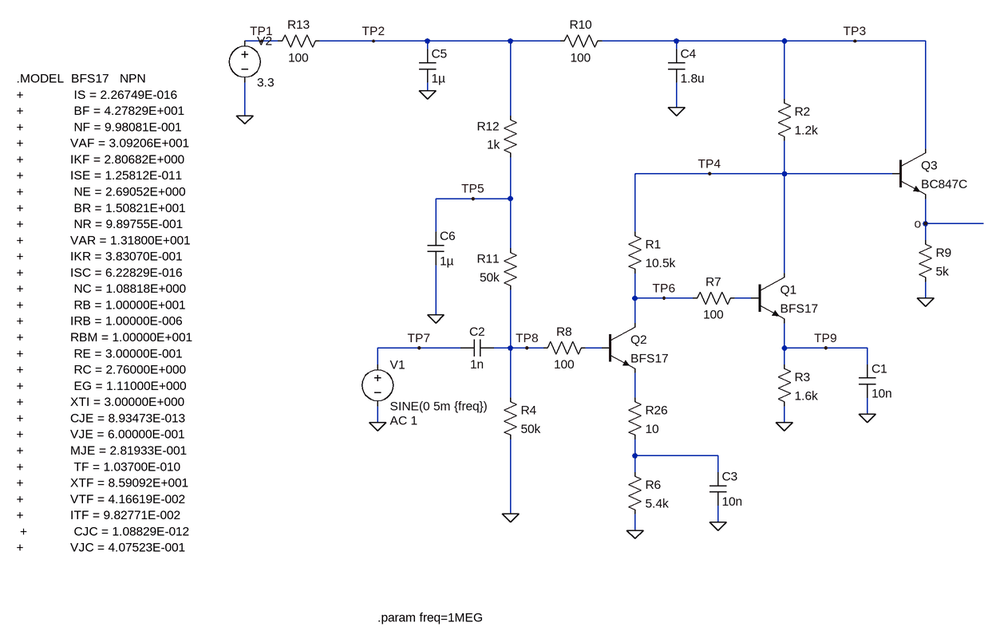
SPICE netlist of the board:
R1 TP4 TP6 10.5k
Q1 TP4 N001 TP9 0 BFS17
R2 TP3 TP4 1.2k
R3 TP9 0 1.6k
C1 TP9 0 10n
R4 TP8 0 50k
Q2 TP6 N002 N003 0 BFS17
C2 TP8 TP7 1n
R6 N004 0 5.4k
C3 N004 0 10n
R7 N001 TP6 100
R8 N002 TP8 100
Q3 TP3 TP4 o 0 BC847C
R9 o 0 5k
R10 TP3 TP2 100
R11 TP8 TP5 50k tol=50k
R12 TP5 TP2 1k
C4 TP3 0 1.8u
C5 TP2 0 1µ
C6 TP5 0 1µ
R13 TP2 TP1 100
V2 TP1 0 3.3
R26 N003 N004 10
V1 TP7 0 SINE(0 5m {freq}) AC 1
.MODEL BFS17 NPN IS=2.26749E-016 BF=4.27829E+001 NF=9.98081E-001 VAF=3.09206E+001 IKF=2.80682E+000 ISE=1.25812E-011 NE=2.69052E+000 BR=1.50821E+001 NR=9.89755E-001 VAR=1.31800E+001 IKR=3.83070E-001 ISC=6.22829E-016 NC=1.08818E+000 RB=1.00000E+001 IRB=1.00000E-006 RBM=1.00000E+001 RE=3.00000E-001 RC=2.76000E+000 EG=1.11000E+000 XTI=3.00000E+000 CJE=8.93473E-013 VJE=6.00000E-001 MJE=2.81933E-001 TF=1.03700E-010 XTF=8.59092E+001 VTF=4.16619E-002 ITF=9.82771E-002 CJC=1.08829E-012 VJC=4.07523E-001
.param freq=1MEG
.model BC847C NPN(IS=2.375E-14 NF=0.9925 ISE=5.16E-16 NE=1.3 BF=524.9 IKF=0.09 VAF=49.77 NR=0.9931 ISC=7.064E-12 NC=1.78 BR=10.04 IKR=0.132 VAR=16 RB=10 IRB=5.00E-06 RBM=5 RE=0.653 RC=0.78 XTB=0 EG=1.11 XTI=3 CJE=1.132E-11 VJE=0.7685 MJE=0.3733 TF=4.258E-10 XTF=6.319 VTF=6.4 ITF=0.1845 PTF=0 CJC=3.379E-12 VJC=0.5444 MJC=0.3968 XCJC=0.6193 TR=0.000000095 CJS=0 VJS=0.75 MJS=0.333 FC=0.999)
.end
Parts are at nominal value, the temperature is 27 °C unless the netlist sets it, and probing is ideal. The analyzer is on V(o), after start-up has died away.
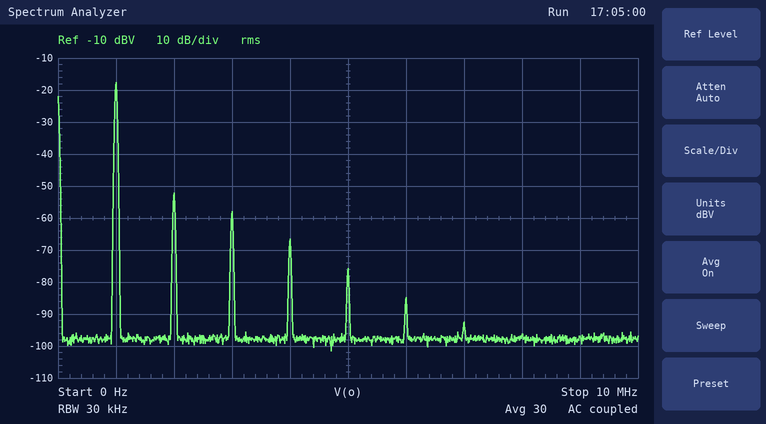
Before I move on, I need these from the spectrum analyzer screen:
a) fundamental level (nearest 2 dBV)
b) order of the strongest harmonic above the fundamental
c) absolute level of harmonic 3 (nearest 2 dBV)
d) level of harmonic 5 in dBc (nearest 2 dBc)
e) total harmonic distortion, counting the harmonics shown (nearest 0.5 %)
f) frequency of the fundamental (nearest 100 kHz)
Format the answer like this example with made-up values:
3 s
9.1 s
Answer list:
-18 dBV
2
-58 dBV
-58 dBc
2.0 %
1.0 MHz
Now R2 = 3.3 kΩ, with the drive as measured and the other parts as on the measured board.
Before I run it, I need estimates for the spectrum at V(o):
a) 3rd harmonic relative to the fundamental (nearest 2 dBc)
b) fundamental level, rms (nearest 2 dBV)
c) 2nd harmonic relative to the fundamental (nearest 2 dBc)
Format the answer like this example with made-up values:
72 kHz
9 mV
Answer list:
-34 dBc
-18 dBV
-28 dBc
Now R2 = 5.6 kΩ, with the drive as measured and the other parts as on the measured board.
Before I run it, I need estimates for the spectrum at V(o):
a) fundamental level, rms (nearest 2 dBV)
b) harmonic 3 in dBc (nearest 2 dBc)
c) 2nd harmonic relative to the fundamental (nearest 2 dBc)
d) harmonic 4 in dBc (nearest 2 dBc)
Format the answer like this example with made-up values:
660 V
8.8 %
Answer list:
-22 dBV
-38 dBc
-20 dBc
-54 dBc
